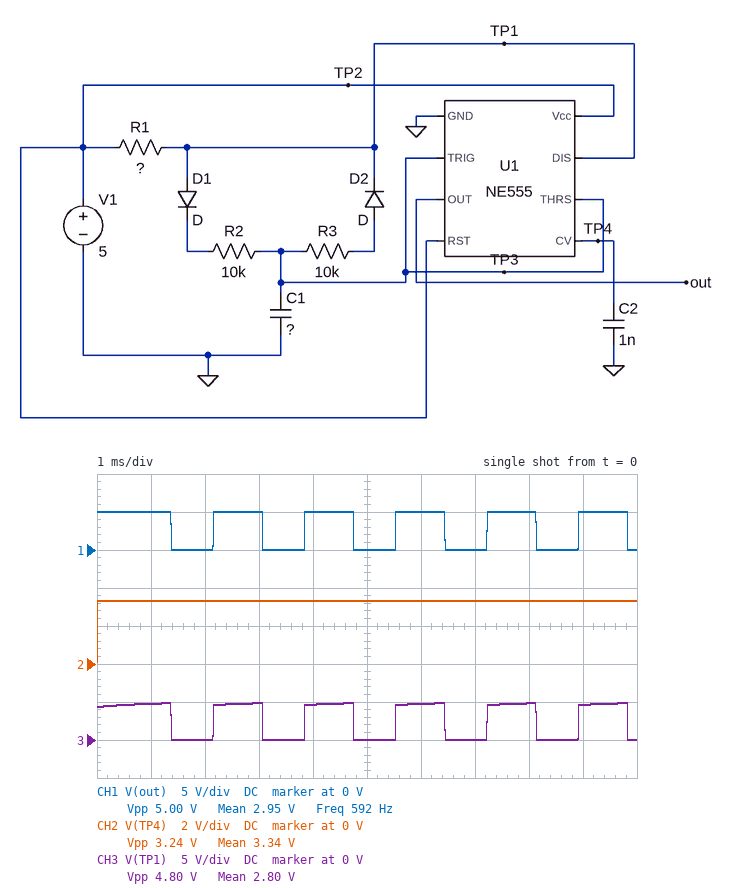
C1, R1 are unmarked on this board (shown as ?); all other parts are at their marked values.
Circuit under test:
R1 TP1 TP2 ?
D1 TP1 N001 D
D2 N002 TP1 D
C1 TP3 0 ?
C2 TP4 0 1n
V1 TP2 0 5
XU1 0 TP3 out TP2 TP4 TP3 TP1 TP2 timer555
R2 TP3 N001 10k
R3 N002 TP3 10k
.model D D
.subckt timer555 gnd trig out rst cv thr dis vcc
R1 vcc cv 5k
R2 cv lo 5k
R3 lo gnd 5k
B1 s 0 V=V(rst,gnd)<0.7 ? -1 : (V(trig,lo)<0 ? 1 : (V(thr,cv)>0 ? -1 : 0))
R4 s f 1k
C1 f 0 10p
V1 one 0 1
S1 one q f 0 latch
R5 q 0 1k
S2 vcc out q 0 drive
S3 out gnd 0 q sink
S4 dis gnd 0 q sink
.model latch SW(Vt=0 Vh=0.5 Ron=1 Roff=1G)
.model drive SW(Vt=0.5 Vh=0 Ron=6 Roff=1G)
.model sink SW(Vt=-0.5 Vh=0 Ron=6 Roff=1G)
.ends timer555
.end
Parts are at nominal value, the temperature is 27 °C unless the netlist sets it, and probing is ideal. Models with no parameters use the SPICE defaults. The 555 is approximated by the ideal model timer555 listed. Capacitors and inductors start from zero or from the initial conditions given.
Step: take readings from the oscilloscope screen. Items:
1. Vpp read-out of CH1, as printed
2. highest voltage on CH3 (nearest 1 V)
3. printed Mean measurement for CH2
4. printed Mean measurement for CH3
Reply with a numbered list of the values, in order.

1. 5.00 V
2. 5 V
3. 3.34 V
4. 2.80 V
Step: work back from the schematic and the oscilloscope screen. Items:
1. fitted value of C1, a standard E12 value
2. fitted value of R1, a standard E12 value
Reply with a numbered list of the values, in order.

1. 82 nF
2. 1.8 kΩ
